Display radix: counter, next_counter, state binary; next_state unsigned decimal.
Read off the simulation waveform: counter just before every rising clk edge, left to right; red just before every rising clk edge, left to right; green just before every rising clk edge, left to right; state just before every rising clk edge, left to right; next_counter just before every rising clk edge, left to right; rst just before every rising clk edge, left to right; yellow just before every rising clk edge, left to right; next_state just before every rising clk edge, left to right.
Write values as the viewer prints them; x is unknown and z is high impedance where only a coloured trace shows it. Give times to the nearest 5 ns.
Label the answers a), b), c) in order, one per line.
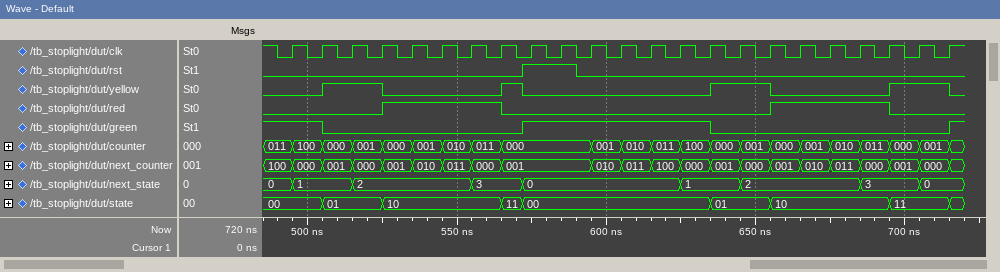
a) 011, 100, 000, 001, 000, 001, 010, 011, 000, 000, 000, 001, 010, 011, 100, 000, 001, 000, 001, 010, 011, 000, 001
b) 0 0 0 0 1 1 1 1 0 0 0 0 0 0 0 0 0 1 1 1 1 0 0
c) 1 1 0 0 0 0 0 0 1 1 1 1 1 1 1 0 0 0 0 0 0 0 0
d) 00, 00, 01, 01, 10, 10, 10, 10, 00, 00, 00, 00, 00, 00, 00, 01, 01, 10, 10, 10, 10, 11, 11
e) 100, 000, 001, 000, 001, 010, 011, 000, 001, 001, 001, 010, 011, 100, 000, 001, 000, 001, 010, 011, 000, 001, 000
f) 0 0 0 0 0 0 0 0 1 1 0 0 0 0 0 0 0 0 0 0 0 0 0
g) 0 0 1 1 0 0 0 0 0 0 0 0 0 0 0 1 1 0 0 0 0 1 1
h) 0, 1, 1, 2, 2, 2, 2, 3, 0, 0, 0, 0, 0, 0, 1, 1, 2, 2, 2, 2, 3, 3, 0
